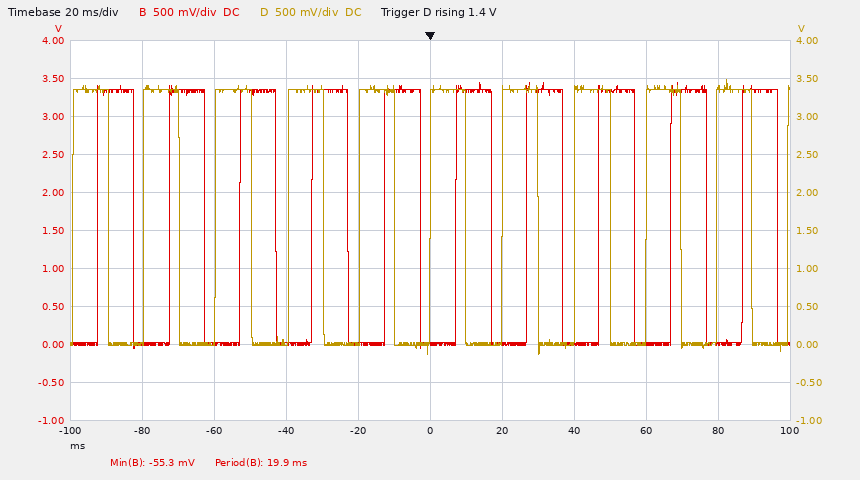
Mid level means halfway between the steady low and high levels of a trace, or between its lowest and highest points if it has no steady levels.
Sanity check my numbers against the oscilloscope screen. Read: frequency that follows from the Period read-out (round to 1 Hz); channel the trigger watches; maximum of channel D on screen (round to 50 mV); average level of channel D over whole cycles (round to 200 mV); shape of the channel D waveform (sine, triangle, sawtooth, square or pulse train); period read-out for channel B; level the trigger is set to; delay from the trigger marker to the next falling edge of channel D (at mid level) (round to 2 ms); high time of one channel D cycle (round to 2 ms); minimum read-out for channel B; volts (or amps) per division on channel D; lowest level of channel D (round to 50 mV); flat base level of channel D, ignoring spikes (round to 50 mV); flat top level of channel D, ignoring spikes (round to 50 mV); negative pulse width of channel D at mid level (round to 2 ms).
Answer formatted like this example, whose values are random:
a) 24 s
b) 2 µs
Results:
a) 50 Hz
b) channel D
c) 3.50 V
d) 1.6 V
e) square
f) 19.9 ms
g) 1.4 V
h) 10 ms
i) 10 ms
j) -55.3 mV
k) 500 mV
l) -150 mV
m) 0 mV
n) 3.35 V
o) 10 ms
